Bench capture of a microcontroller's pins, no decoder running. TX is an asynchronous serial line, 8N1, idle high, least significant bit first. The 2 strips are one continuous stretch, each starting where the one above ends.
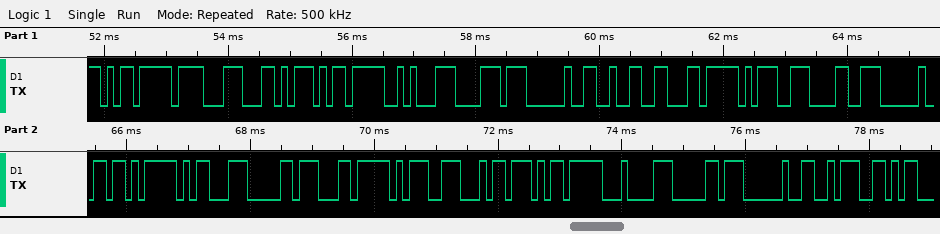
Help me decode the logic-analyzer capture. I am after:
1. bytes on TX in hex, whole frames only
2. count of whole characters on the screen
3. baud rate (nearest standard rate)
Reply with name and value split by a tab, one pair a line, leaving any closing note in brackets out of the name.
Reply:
bytes on TX in hex, whole frames only	ED 8F AC ED 8A B8 20 32 EC 9D 98 20 EB 8D B0 EC 9D B4 ED 84 B0 20 3A
count of whole characters on the screen	23
baud rate	9600 baud
